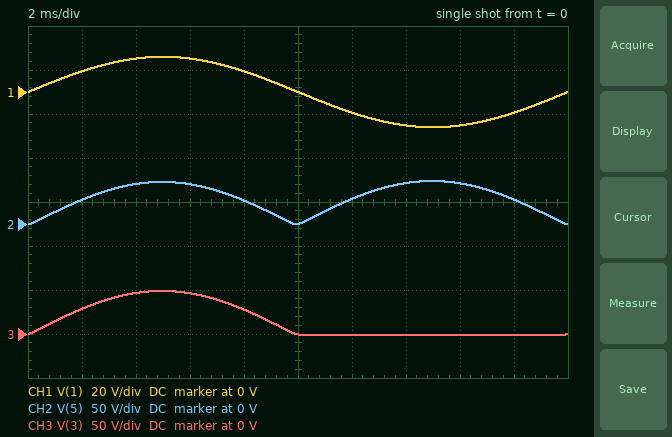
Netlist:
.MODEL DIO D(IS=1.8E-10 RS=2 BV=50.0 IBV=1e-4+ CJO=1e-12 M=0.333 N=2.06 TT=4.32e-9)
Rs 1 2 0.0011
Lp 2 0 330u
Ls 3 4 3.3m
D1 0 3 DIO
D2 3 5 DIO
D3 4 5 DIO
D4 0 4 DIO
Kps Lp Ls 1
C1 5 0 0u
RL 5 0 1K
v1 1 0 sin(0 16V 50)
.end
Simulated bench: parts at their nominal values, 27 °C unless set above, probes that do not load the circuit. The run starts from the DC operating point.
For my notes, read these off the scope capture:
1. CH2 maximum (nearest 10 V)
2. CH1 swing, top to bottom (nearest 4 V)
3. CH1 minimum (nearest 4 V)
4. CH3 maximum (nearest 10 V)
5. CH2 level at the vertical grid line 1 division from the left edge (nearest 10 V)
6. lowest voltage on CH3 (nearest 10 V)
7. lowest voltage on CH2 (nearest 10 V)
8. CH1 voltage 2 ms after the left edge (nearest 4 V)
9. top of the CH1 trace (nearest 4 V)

50 V
32 V
-16 V
50 V
30 V
0 V
0 V
8 V
16 V
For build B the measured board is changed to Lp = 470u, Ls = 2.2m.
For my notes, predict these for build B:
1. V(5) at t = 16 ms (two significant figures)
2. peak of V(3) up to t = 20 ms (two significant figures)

31 V
33 V
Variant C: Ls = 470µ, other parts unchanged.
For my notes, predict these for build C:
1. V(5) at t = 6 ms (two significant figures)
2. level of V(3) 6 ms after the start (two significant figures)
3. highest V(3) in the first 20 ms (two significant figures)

16 V
17 V
18 V
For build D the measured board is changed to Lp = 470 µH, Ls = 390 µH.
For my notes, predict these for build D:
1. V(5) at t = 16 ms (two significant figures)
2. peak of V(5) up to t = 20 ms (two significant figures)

12 V
13 V
